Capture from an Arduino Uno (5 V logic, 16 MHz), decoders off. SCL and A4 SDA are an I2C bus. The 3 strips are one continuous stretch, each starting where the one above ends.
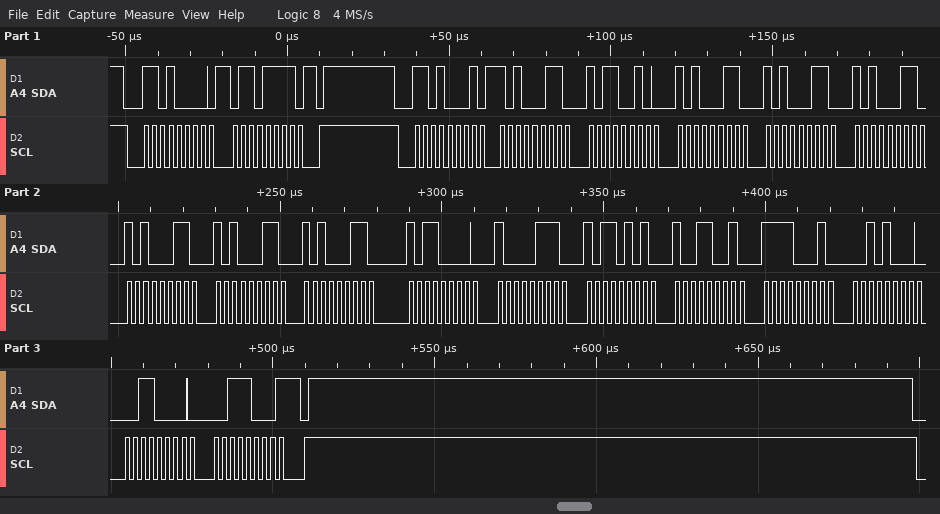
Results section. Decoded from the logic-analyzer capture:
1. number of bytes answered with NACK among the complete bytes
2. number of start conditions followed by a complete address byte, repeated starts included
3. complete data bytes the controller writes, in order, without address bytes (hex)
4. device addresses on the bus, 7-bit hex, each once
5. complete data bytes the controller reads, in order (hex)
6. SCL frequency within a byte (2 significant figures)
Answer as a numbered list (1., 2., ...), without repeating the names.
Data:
1. 1
2. 2
3. 6F
4. 0x68
5. A3 B2 A3 A3 A3 A3 A3 A3 B0 87 B5 99 F1 28 30 38
6. 400 kHz
